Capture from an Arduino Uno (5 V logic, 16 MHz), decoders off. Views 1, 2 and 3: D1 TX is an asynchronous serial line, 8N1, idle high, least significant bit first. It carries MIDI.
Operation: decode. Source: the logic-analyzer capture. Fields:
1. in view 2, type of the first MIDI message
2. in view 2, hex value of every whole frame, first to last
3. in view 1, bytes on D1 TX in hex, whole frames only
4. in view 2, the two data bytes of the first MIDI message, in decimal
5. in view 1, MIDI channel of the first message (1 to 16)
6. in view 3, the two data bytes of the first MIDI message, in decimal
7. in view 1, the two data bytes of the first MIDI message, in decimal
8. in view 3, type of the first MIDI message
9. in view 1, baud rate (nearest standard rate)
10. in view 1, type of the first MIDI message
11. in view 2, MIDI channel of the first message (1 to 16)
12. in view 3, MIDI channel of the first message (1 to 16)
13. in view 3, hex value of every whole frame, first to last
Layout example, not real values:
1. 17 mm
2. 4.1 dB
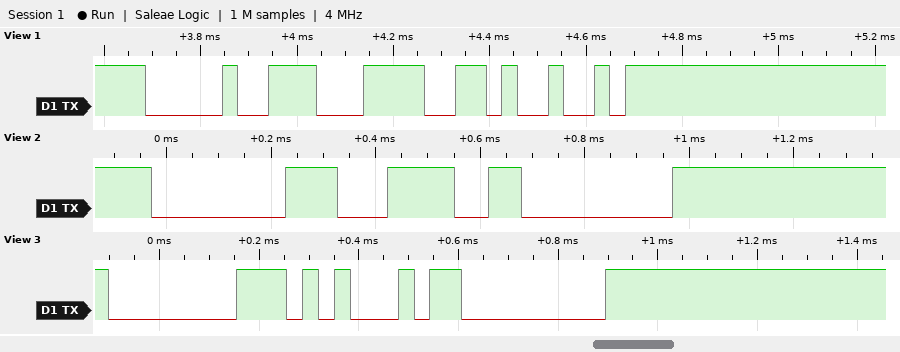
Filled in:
1. Note Off
2. 0x80 0x3C 0x00
3. 0x90 0x3C 0x49
4. 60, 0
5. 1
6. 69, 0
7. 60, 73
8. Note Off
9. 31250 baud
10. Note On
11. 1
12. 1
13. 0x80 0x45 0x00
